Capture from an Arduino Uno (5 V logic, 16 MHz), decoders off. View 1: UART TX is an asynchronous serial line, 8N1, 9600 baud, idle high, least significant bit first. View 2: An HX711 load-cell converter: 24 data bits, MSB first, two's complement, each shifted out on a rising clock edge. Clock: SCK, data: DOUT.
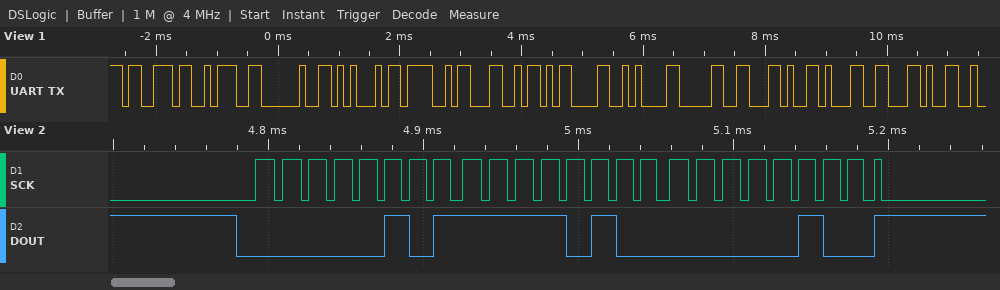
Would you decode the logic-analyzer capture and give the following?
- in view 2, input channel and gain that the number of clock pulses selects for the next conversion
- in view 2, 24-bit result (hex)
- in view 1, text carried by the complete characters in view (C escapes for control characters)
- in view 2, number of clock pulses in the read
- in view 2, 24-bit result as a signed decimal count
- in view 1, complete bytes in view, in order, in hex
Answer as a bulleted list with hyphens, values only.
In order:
- channel A, gain 128
- 0x05F404
- "s: EOL\r\n0,1,"
- 25
- 390148
- 0x73 0x3A 0x20 0x45 0x4F 0x4C 0x0D 0x0A 0x30 0x2C 0x31 0x2C
